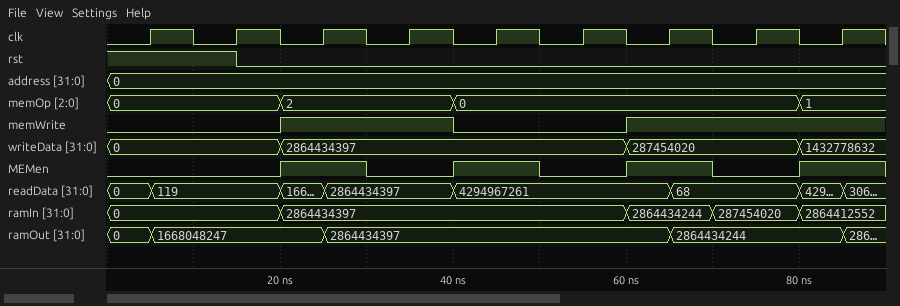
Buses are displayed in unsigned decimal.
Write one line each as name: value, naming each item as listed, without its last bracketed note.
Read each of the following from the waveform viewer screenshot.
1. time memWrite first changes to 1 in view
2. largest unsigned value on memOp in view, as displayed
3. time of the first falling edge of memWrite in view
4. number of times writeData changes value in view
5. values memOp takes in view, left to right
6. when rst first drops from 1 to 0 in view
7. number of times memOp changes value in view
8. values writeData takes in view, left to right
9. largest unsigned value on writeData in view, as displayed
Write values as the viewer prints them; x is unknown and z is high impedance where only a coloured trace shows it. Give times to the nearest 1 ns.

time memWrite first changes to 1 in view: 20 ns
largest unsigned value on memOp in view, as displayed: 2
time of the first falling edge of memWrite in view: 40 ns
number of times writeData changes value in view: 3
values memOp takes in view, left to right: 0, 2, 0, 1
when rst first drops from 1 to 0 in view: 15 ns
number of times memOp changes value in view: 3
values writeData takes in view, left to right: 0, 2864434397, 287454020, 1432778632
largest unsigned value on writeData in view, as displayed: 2864434397
